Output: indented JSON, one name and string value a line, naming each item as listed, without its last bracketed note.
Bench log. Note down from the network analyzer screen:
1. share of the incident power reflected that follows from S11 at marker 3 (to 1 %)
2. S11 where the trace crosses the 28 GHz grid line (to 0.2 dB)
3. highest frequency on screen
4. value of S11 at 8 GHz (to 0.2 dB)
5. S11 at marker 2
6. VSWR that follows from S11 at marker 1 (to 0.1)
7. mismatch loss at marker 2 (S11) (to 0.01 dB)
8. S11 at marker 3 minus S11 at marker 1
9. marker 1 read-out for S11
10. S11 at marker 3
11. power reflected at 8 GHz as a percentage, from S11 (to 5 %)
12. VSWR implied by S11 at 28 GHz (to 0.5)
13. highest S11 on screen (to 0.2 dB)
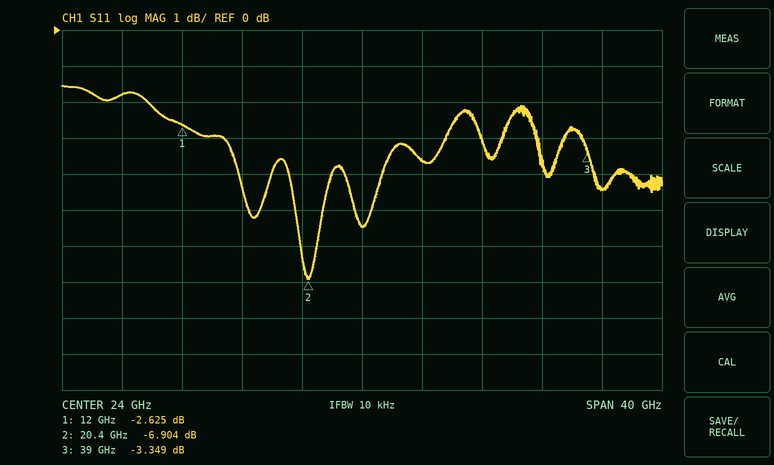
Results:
{
  "share of the incident power reflected that follows from S11 at marker 3": "46 %",
  "S11 where the trace crosses the 28 GHz grid line": "-3.6 dB",
  "highest frequency on screen": "44 GHz",
  "value of S11 at 8 GHz": "-1.8 dB",
  "S11 at marker 2": "-6.904 dB",
  "VSWR that follows from S11 at marker 1": "6.7",
  "mismatch loss at marker 2 (S11)": "0.99 dB",
  "S11 at marker 3 minus S11 at marker 1": "-0.724 dB",
  "marker 1 read-out for S11": "-2.625 dB",
  "S11 at marker 3": "-3.349 dB",
  "power reflected at 8 GHz as a percentage, from S11": "65 %",
  "VSWR implied by S11 at 28 GHz": "5.0",
  "highest S11 on screen": "-1.6 dB"
}
